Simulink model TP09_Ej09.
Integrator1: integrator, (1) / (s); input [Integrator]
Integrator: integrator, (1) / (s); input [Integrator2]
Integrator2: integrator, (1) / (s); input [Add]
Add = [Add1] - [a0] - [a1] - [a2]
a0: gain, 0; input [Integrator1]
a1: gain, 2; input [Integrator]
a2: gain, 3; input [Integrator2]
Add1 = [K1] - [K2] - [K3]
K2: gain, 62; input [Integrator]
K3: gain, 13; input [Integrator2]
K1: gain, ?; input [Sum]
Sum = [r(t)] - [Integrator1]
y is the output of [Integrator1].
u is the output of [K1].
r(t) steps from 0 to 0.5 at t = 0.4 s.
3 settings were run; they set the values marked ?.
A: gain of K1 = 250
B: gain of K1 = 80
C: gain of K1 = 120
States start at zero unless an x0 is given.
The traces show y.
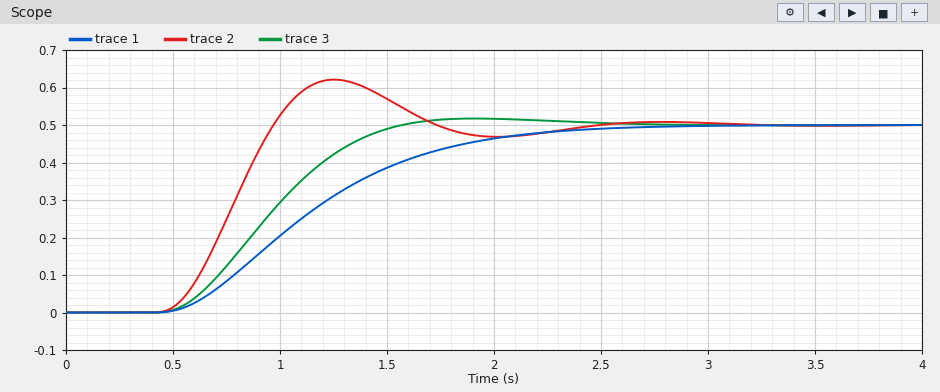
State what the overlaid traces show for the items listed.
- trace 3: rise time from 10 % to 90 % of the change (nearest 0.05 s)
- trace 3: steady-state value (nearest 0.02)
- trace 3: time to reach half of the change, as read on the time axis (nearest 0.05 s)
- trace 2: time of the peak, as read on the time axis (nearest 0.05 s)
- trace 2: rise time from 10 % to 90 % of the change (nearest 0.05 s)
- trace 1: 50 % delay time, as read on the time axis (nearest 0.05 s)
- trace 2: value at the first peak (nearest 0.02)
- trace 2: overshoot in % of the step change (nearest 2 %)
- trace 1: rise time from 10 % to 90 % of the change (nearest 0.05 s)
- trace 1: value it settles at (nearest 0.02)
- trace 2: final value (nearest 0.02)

0.70 s
0.50
0.95 s
1.25 s
0.35 s
1.10 s
0.62
24 %
1.20 s
0.50
0.50
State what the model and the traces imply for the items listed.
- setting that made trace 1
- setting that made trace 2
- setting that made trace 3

B
A
C
